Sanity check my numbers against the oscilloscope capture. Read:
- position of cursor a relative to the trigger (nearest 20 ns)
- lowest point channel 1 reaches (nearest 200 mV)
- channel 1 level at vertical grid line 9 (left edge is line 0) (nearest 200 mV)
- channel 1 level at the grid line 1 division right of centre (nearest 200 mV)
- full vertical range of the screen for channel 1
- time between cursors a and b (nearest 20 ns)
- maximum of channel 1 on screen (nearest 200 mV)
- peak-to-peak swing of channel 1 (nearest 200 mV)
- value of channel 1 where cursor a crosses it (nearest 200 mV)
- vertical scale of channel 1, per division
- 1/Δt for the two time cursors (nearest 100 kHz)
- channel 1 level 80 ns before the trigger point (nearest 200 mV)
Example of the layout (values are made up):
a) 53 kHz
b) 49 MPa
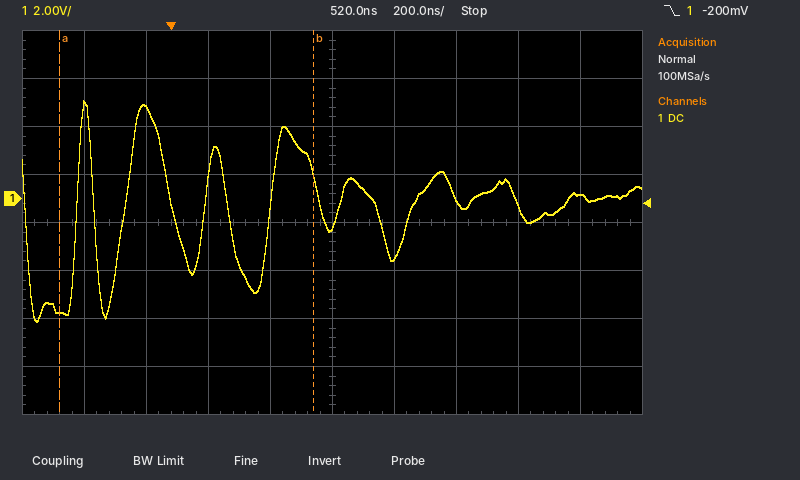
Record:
a) -360 ns
b) -5.2 V
c) 200 mV
d) -2.4 V
e) 16 V
f) 820 ns
g) 4.0 V
h) 9.2 V
i) -4.8 V
j) 2 V
k) 1.2 MHz
l) 3.8 V
